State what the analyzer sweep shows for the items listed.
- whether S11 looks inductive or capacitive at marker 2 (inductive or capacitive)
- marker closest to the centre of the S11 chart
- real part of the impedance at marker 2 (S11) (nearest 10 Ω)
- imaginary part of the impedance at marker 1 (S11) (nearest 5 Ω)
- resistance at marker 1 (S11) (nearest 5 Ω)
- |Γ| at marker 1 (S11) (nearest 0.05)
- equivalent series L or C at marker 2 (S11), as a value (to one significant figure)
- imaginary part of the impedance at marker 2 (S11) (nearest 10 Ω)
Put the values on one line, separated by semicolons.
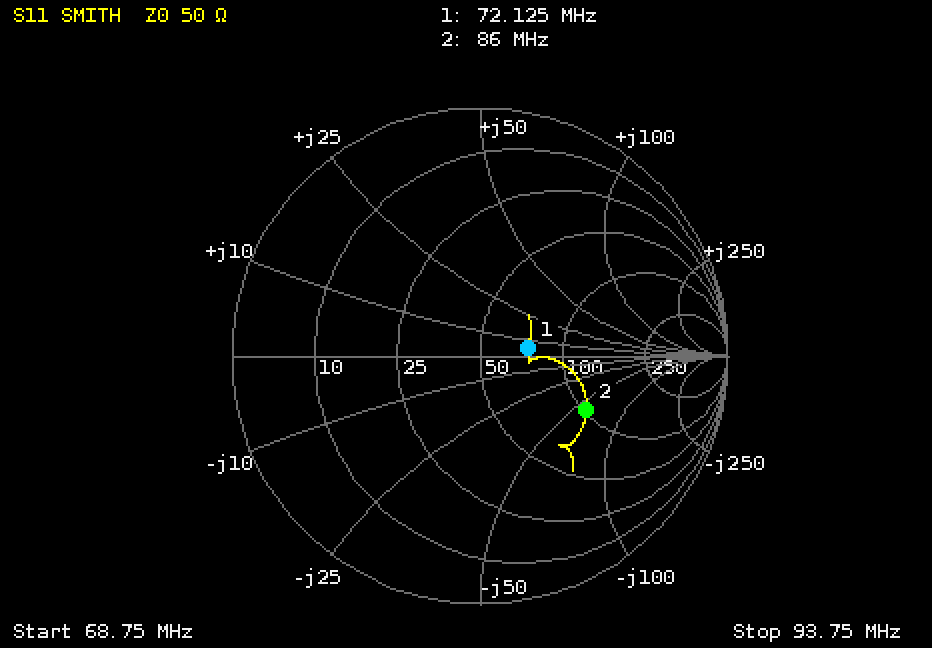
capacitive; marker 1; 100 Ω; +5 Ω; 75 Ω; 0.20; 30 pF; -60 Ω
